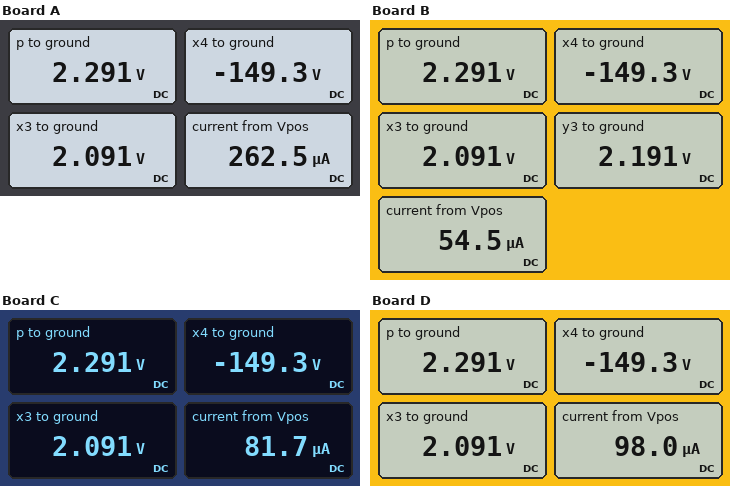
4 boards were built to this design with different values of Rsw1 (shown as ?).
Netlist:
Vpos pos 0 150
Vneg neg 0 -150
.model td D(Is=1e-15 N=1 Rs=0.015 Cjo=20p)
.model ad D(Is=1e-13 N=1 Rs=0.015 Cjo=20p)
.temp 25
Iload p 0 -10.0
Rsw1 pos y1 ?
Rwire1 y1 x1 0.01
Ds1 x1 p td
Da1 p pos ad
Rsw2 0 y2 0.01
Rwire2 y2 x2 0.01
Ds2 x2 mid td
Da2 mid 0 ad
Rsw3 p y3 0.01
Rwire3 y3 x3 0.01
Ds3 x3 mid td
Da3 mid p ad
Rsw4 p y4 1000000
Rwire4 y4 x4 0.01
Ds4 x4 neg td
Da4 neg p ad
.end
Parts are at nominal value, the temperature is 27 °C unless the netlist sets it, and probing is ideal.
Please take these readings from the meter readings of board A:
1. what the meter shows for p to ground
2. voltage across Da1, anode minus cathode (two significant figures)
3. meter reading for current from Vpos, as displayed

2.291 V
-150 V
262.5 µA
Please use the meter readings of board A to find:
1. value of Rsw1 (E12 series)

560 kΩ
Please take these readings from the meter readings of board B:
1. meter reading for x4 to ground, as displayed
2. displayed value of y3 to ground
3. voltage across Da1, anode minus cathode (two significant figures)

-149.3 V
2.191 V
-150 V
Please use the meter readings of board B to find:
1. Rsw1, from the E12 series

2.7 MΩ
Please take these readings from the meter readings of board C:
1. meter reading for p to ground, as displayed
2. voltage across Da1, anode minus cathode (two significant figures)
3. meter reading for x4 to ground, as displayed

2.291 V
-150 V
-149.3 V
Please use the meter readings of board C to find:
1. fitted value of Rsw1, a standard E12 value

1.8 MΩ
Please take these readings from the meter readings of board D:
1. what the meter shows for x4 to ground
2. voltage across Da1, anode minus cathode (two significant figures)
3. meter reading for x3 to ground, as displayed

-149.3 V
-150 V
2.091 V
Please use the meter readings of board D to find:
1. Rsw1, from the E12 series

1.5 MΩ
